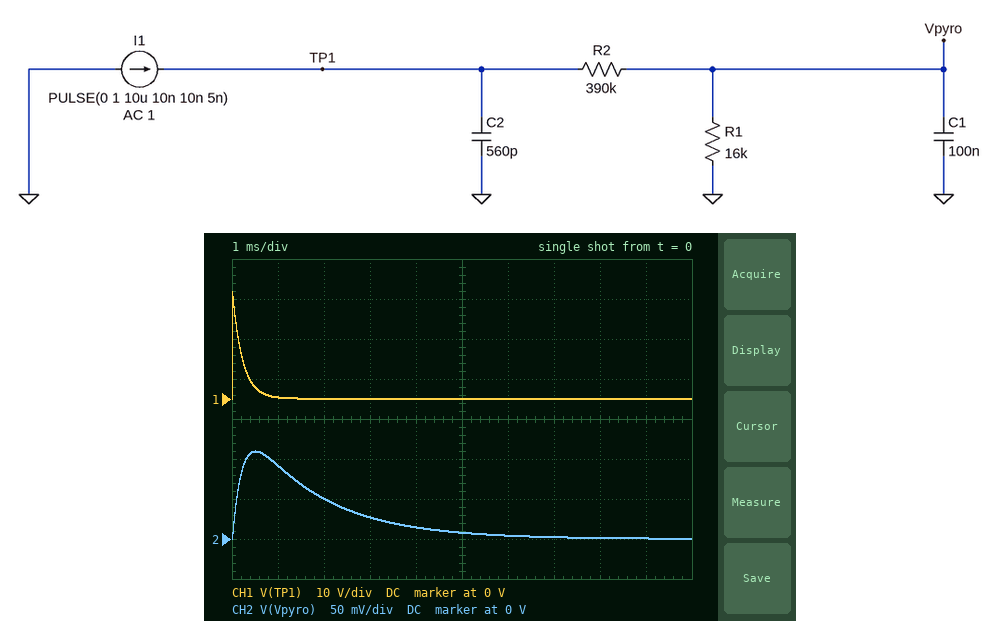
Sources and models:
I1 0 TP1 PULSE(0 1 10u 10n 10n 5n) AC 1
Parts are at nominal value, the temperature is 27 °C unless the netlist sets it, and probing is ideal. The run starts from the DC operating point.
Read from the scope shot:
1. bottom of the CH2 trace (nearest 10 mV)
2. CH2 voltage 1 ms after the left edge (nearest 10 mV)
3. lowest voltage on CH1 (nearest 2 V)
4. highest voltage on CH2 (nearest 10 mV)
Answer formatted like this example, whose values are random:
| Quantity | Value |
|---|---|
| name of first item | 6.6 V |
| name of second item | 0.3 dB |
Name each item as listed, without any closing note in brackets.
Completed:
| Quantity | Value |
|---|---|
| bottom of the CH2 trace | 0 V |
| CH2 voltage 1 ms after the left edge | 90 mV |
| lowest voltage on CH1 | 0 V |
| highest voltage on CH2 | 110 mV |
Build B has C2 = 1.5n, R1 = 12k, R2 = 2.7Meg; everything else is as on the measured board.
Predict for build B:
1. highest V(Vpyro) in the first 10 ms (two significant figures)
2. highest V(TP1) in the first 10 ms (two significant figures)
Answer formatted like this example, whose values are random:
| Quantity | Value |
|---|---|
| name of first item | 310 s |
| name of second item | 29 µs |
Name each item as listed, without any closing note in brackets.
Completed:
| Quantity | Value |
|---|---|
| highest V(Vpyro) in the first 10 ms | 27 mV |
| highest V(TP1) in the first 10 ms | 10 V |
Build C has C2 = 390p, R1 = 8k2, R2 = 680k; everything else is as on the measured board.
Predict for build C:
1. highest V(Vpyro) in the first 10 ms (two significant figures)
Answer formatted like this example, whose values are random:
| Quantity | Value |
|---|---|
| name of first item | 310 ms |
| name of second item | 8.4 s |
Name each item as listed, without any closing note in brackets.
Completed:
| Quantity | Value |
|---|---|
| highest V(Vpyro) in the first 10 ms | 88 mV |
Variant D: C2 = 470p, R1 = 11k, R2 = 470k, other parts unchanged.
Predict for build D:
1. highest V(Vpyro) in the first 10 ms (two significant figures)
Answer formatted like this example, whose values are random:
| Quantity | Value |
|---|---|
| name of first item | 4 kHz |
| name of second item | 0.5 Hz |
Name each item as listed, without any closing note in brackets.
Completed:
| Quantity | Value |
|---|---|
| highest V(Vpyro) in the first 10 ms | 100 mV |
